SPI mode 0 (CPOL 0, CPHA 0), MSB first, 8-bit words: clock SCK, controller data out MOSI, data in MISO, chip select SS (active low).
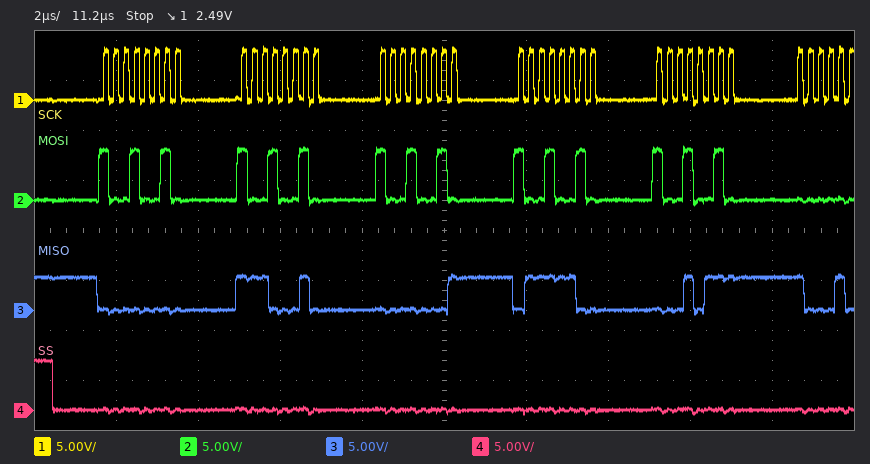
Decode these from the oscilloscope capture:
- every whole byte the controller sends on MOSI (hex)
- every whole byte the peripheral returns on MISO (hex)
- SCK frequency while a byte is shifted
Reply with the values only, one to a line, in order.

0x92 0x92 0x92 0x92 0x92
0x00 0xE2 0x01 0x7C 0x17
4 MHz
